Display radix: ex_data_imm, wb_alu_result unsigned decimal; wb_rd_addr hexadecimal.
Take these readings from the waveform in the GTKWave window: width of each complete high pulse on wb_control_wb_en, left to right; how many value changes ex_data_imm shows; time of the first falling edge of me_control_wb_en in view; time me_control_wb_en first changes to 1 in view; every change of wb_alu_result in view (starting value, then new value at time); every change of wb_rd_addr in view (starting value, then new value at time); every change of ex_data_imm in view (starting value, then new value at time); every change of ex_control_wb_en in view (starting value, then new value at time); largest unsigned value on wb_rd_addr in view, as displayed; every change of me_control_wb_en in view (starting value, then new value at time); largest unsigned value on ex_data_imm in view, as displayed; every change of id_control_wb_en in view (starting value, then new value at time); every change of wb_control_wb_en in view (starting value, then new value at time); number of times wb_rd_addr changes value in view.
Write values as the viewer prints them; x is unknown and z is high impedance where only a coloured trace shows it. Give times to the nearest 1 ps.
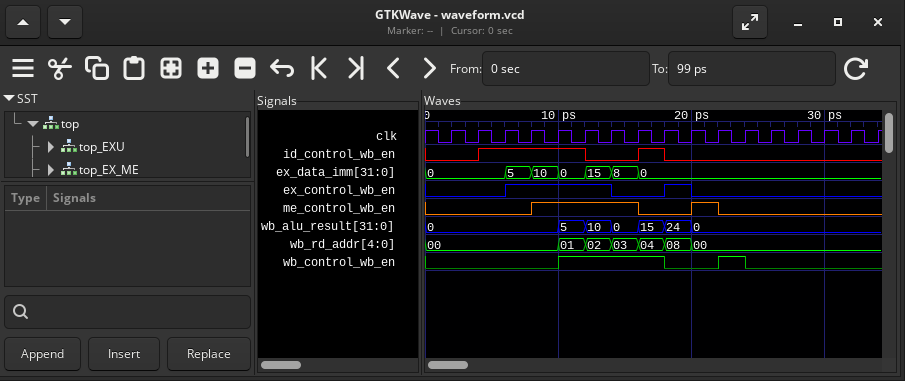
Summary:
8 ps, 2 ps
6
16 ps
8 ps
0, 5 at 10 ps, 10 at 12 ps, 0 at 14 ps, 15 at 16 ps, 24 at 18 ps, 0 at 20 ps
00, 01 at 10 ps, 02 at 12 ps, 03 at 14 ps, 04 at 16 ps, 08 at 18 ps, 00 at 20 ps
0, 5 at 6 ps, 10 at 8 ps, 0 at 10 ps, 15 at 12 ps, 8 at 14 ps, 0 at 16 ps
0, 1 at 6 ps, 0 at 14 ps, 1 at 18 ps, 0 at 20 ps
08
0, 1 at 8 ps, 0 at 16 ps, 1 at 20 ps, 0 at 22 ps
15
0, 1 at 4 ps, 0 at 12 ps, 1 at 16 ps, 0 at 18 ps
0, 1 at 10 ps, 0 at 18 ps, 1 at 22 ps, 0 at 24 ps
6
